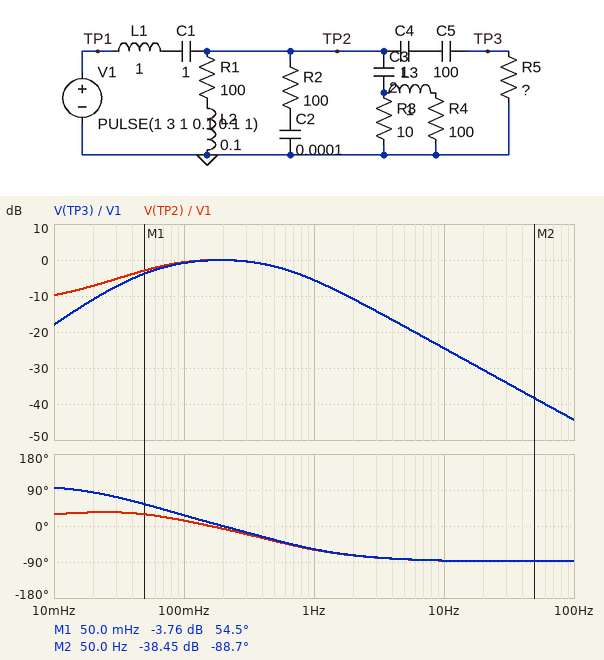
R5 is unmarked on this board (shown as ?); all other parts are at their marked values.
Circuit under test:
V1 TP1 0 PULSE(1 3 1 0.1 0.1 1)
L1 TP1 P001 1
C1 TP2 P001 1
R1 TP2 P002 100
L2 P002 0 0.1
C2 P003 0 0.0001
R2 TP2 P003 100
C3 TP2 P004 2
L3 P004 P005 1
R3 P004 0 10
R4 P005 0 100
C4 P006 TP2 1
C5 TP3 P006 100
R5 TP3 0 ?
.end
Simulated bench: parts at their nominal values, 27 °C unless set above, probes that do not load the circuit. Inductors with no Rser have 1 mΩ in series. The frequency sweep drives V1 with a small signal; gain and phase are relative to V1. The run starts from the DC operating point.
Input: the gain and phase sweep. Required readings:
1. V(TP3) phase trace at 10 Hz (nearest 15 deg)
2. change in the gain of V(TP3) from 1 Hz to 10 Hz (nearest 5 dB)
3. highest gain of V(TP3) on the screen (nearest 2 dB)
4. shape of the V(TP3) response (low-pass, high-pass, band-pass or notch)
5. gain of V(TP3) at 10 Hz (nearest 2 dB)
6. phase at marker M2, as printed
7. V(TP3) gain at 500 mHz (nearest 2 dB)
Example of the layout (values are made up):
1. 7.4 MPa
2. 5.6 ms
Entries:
1. -90 deg
2. -20 dB
3. 0 dB
4. band-pass
5. -24 dB
6. -88.7 deg
7. -2 dB
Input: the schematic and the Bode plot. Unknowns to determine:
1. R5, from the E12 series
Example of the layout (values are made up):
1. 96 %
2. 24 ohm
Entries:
1. 6.8 Ω
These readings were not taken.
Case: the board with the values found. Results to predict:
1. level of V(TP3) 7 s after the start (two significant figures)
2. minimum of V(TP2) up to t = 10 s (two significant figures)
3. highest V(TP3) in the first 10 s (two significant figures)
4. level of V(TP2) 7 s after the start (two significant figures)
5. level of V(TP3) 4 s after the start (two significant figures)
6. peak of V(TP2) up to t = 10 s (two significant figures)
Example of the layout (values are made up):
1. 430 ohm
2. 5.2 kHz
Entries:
1. -120 mV
2. -390 mV
3. 1.6 V
4. -99 mV
5. -460 mV
6. 1.8 V
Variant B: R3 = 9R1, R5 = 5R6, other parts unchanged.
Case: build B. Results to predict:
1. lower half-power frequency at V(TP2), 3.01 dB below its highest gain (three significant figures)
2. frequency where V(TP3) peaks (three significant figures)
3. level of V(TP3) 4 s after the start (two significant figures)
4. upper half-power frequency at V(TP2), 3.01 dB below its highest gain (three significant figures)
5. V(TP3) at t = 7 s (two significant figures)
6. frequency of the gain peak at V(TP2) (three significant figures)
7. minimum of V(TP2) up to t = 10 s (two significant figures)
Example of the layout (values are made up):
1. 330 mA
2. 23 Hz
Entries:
1. 55.5 mHz
2. 193 mHz
3. -500 mV
4. 573 mHz
5. -94 mV
6. 185 mHz
7. -420 mV
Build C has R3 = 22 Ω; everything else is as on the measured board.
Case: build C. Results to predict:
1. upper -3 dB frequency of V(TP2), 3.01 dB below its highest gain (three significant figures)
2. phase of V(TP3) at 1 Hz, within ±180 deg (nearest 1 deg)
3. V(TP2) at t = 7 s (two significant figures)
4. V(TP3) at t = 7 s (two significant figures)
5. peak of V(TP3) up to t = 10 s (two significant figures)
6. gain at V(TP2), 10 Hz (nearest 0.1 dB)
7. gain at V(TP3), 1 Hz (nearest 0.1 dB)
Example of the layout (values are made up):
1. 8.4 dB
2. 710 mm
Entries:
1. 792 mHz
2. -52 deg
3. -100 mV
4. -140 mV
5. 1.7 V
6. -22.5 dB
7. -4.2 dB
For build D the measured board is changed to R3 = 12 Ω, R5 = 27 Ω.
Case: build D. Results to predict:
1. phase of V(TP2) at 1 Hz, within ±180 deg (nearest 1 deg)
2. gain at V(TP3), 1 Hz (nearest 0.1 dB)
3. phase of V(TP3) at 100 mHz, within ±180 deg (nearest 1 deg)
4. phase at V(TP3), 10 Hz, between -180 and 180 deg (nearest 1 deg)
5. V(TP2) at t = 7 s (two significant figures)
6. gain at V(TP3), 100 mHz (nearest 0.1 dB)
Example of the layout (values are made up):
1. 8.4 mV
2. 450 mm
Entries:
1. -41 deg
2. -2.4 dB
3. 11 deg
4. -83 deg
5. -120 mV
6. -0.2 dB
